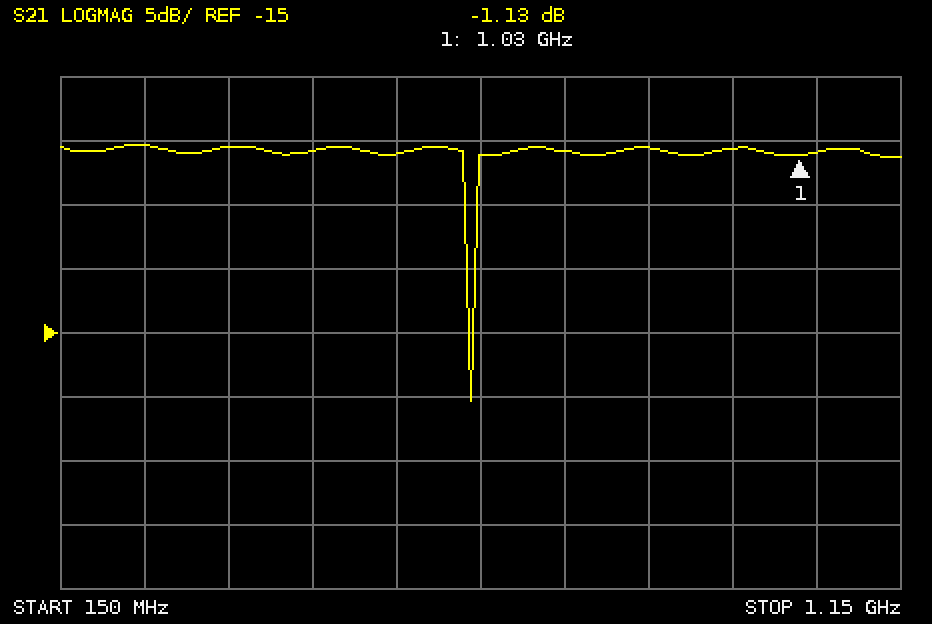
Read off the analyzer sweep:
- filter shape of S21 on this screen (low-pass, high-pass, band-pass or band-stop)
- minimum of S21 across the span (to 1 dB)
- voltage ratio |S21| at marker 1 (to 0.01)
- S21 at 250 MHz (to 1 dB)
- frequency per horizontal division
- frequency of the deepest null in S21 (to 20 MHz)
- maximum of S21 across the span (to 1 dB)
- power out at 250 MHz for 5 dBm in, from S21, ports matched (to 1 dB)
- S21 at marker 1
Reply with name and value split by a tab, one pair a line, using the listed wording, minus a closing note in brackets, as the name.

filter shape of S21 on this screen	band-stop
minimum of S21 across the span	-20 dB
voltage ratio |S21| at marker 1	0.88
S21 at 250 MHz	0 dB
frequency per horizontal division	100 MHz
frequency of the deepest null in S21	640 MHz
maximum of S21 across the span	0 dB
power out at 250 MHz for 5 dBm in, from S21, ports matched	5 dBm
S21 at marker 1	-1.13 dB
